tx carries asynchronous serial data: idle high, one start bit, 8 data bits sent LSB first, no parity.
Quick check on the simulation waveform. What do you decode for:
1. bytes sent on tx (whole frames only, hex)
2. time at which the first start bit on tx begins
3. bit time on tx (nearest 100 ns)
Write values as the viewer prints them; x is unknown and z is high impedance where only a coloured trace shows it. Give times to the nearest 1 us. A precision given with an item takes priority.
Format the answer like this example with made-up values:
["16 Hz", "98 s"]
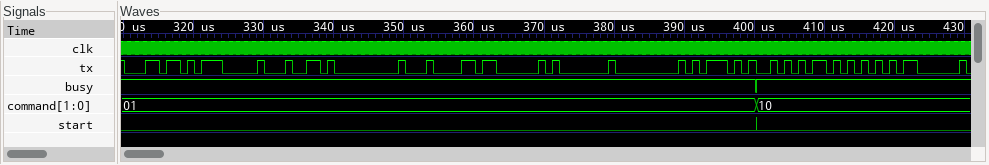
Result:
["6C, 07, 64, 00, 84, 03, 01, 00, 5D, AA, 55, 03", "310 us", "1000 ns"]
